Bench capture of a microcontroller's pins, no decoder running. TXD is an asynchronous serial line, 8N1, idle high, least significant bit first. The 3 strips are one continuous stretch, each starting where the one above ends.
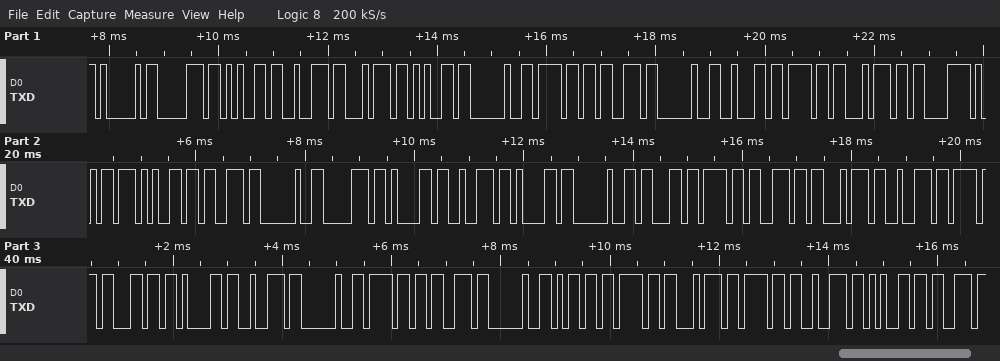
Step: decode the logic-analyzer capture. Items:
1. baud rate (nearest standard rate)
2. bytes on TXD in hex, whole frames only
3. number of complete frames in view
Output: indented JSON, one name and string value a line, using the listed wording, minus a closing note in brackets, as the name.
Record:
{
  "baud rate": "9600 baud",
  "bytes on TXD in hex, whole frames only": "41 70 65 72 74 65 20 6F 73 20 62 6F 74 C3 B5 65 73 20 70 61 72 61 20 63 6F 6E 74 72 6F 6C 61 72 20 6F 73 20 6D 6F 74 6F 72 65 73",
  "number of complete frames in view": "43"
}
